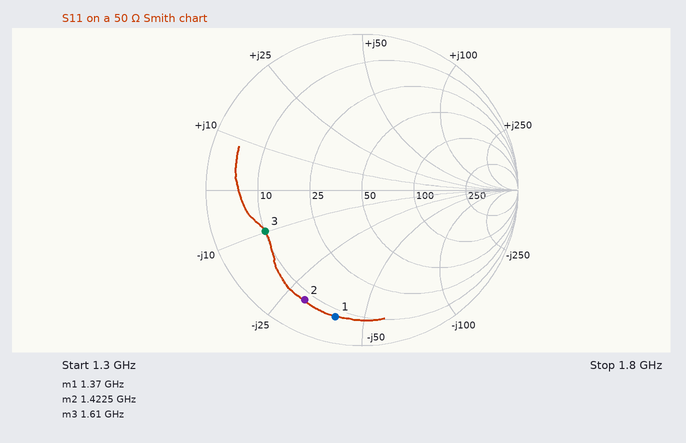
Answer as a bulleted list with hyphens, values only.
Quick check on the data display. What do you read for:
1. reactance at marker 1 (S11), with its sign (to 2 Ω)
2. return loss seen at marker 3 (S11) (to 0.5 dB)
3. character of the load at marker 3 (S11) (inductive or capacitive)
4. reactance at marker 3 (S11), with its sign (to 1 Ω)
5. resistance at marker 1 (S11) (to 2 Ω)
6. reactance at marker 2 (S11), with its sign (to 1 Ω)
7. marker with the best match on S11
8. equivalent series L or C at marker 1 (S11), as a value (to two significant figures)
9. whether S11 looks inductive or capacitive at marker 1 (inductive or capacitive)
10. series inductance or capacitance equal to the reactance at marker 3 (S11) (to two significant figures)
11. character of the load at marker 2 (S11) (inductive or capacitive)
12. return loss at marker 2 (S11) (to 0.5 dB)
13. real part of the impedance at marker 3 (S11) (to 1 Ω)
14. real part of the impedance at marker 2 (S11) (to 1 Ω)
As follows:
- -40 Ω
- 3.5 dB
- capacitive
- -10 Ω
- 8 Ω
- -30 Ω
- marker 3
- 2.9 pF
- capacitive
- 10 pF
- capacitive
- 2.0 dB
- 10 Ω
- 8 Ω
